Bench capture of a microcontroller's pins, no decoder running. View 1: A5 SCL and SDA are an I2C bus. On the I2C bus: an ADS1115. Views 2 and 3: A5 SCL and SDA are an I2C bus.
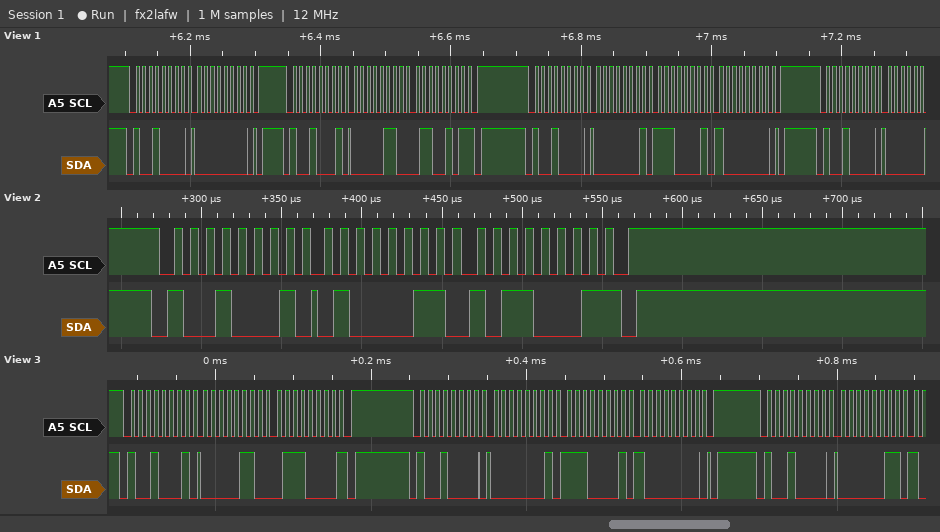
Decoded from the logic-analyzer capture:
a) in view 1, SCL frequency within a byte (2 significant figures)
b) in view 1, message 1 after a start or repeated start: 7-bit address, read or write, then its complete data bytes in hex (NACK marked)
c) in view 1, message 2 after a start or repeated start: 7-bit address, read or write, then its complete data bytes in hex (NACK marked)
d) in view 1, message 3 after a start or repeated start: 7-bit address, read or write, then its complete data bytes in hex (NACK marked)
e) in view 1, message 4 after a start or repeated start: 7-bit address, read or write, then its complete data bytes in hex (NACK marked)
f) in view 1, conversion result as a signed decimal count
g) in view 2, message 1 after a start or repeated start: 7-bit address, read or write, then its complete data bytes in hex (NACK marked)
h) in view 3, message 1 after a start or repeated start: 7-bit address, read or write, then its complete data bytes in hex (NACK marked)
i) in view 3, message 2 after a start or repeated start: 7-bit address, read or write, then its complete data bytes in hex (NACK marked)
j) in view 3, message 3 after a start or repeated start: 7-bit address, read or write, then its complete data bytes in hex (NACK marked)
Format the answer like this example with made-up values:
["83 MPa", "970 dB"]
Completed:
["100 kHz", "0x48 write: 00", "0x48 read: 06 65 NACK", "0x48 write: 01 E1 80", "0x48 write", "1637", "0x48 read: 43 B1 NACK", "0x48 read: 06 70 NACK", "0x48 write: 01 E1 80", "0x48 write: 03"]
